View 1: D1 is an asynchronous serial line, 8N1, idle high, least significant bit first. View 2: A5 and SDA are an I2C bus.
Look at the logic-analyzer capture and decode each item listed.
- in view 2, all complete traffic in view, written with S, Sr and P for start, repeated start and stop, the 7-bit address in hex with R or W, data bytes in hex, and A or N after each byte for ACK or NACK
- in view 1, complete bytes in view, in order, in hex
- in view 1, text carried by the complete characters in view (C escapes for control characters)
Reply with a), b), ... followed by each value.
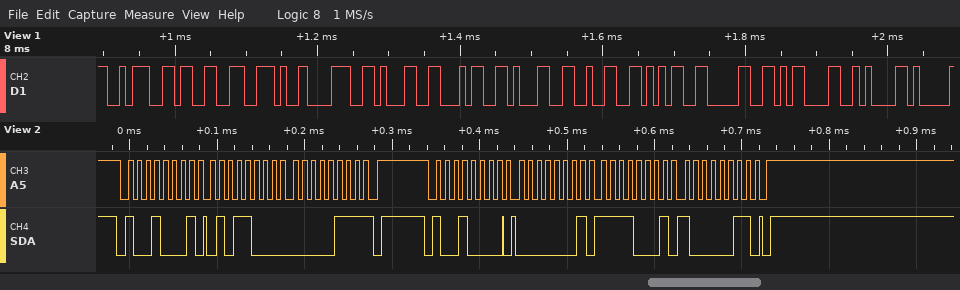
a) S 48R A 58 A 07 N P S 48W A 01 A F1 A 83 A P
b) 3A 33 2E 38 31 34 31 32 35 30 0D 0A
c) ":3.8141250\r\n"
